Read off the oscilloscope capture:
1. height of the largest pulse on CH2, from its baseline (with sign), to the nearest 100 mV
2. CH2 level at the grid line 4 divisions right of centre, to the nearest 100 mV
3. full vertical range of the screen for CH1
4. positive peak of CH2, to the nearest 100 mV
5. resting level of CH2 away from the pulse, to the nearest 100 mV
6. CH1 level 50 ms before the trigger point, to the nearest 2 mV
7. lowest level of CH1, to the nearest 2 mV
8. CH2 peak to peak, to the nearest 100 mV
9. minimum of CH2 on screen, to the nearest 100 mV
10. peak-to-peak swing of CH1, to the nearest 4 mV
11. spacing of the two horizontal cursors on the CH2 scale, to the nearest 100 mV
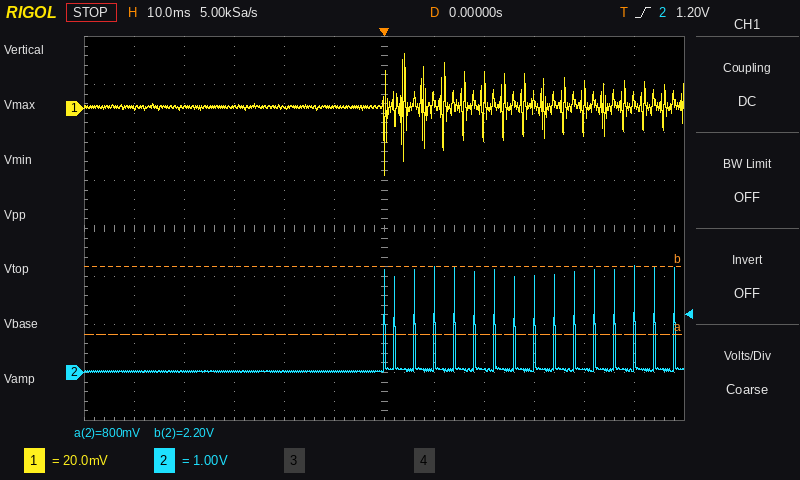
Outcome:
+2.2 V
100 mV
160 mV
2.2 V
0.0 V
0 mV
-28 mV
2.2 V
0.0 V
52 mV
1.4 V
